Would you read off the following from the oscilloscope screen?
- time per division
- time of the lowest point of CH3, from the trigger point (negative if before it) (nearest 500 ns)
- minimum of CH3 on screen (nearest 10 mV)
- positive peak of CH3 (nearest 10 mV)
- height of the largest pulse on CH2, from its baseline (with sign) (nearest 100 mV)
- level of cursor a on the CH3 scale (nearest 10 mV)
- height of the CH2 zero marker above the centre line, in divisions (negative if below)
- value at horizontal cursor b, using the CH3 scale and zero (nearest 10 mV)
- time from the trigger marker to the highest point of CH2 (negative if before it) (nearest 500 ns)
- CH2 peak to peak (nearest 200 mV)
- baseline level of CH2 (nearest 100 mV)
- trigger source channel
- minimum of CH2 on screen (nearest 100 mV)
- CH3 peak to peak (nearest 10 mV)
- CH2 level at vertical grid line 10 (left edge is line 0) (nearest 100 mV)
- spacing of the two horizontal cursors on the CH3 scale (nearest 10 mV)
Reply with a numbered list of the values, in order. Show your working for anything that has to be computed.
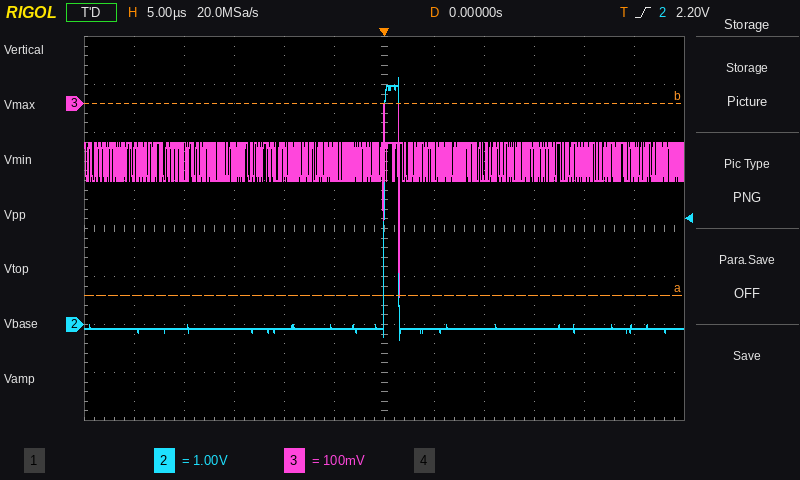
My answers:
1. 5 µs
2. +1.5 µs
3. -400 mV
4. 0 mV
5. +5.2 V
6. -400 mV
7. -2.0 div
8. 0 mV
9. +1.5 µs
10. 5.4 V
11. -100 mV
12. CH2
13. -300 mV
14. 0 mV − (-400 mV) = 400 mV
15. -100 mV
16. 400 mV
